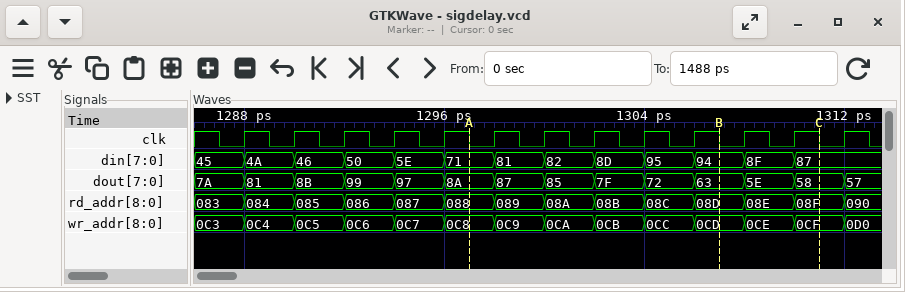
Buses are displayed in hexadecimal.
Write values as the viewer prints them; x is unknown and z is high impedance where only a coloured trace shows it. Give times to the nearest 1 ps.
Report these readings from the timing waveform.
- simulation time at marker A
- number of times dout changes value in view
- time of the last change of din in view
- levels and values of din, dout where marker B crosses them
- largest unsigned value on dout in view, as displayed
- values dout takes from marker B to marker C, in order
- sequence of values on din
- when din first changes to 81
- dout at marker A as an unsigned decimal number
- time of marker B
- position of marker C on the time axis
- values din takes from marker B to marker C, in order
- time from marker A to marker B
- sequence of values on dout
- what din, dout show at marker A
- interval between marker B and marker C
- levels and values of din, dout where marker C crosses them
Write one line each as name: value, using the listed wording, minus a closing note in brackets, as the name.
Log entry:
simulation time at marker A: 1297 ps
number of times dout changes value in view: 13
time of the last change of din in view: 1310 ps
levels and values of din, dout where marker B crosses them: din=94, dout=63
largest unsigned value on dout in view, as displayed: 99
values dout takes from marker B to marker C, in order: 63, 5E, 58
sequence of values on din: 45, 4A, 46, 50, 5E, 71, 81, 82, 8D, 95, 94, 8F, 87
when din first changes to 81: 1298 ps
dout at marker A as an unsigned decimal number: 138
time of marker B: 1307 ps
position of marker C on the time axis: 1311 ps
values din takes from marker B to marker C, in order: 94, 8F, 87
time from marker A to marker B: 10 ps
sequence of values on dout: 7A, 81, 8B, 99, 97, 8A, 87, 85, 7F, 72, 63, 5E, 58, 57
what din, dout show at marker A: din=71, dout=8A
interval between marker B and marker C: 4 ps
levels and values of din, dout where marker C crosses them: din=87, dout=58
